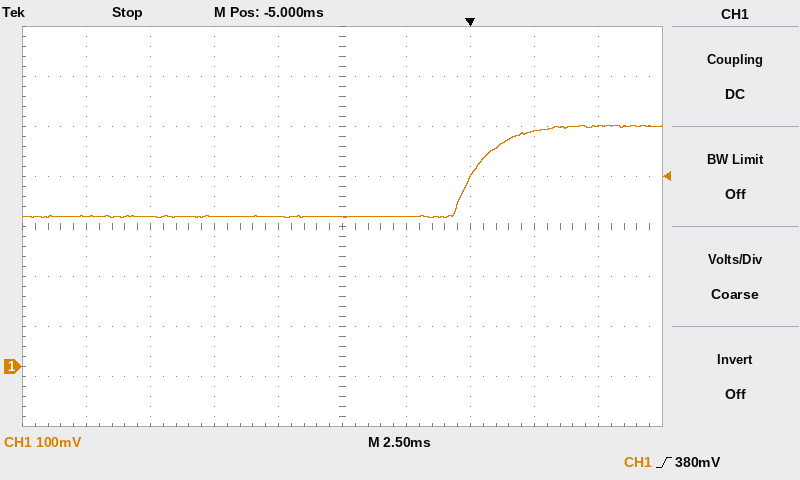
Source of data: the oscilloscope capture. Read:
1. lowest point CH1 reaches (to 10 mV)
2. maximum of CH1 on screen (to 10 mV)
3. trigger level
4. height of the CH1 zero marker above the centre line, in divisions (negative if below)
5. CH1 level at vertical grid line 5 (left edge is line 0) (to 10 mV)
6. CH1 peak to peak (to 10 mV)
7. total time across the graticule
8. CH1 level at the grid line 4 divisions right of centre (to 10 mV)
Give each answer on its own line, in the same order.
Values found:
300 mV
480 mV
380 mV
-2.8 div
300 mV
180 mV
25 ms
480 mV
